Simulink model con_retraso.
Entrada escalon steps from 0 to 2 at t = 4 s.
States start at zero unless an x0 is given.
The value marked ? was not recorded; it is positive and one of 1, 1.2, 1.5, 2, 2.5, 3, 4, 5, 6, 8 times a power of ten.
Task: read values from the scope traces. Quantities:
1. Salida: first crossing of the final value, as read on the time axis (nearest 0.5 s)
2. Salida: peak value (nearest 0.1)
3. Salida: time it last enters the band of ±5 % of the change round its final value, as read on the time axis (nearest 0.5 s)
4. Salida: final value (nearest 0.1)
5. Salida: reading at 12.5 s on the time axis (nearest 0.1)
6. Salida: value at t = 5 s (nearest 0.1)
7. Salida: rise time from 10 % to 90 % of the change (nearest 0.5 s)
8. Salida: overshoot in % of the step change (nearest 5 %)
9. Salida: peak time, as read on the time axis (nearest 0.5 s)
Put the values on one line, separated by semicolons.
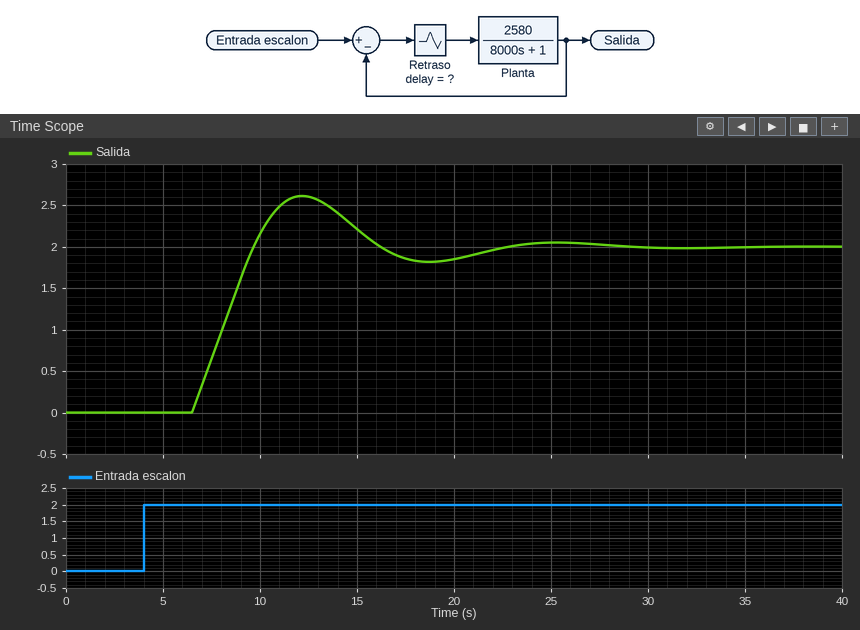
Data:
9.5 s; 2.6; 21.0 s; 2.0; 2.6; 0.0; 2.5 s; 30 %; 12.0 s
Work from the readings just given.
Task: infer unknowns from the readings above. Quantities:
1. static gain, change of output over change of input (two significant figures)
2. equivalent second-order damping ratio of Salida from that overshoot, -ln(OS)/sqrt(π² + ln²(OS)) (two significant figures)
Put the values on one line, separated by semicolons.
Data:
1.0; 0.36
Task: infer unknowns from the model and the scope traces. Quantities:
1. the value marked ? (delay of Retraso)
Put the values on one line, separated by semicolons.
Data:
2.5
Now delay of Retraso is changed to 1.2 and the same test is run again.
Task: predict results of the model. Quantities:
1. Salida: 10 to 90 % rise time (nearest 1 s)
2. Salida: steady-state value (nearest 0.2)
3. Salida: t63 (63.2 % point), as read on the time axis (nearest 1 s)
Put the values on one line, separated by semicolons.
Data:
4 s; 2.0; 7 s
